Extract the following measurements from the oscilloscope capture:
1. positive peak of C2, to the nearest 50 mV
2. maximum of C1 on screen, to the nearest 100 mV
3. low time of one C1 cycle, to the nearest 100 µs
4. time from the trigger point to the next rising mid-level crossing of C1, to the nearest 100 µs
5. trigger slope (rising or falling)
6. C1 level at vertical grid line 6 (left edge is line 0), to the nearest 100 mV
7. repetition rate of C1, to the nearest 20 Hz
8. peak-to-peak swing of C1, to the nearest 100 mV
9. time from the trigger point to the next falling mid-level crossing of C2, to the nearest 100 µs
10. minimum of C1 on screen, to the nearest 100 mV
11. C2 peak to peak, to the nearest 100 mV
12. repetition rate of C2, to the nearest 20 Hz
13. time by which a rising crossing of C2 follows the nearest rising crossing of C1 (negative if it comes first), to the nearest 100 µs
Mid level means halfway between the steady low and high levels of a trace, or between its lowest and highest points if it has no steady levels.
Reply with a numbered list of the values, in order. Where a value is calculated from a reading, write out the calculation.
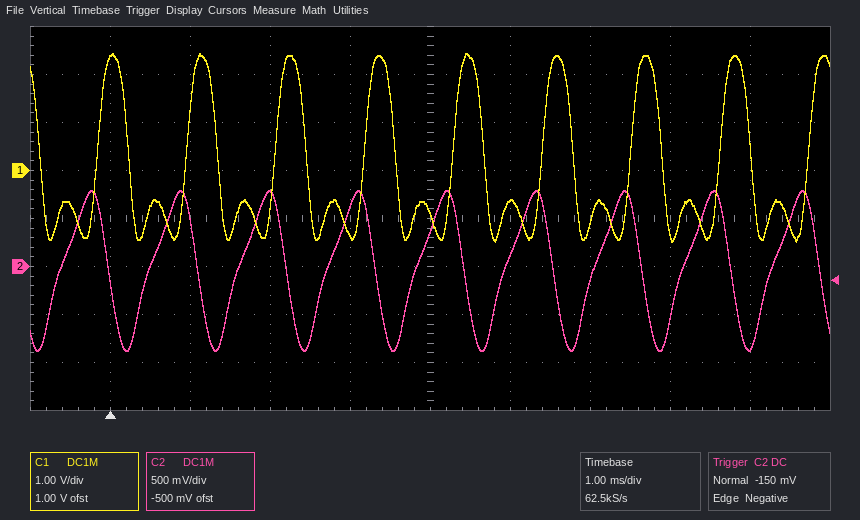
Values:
1. 800 mV
2. 2.4 V
3. 700 µs
4. 1.0 ms
5. falling
6. -700 mV
7. 900 Hz
8. 2.4 V − (-1.5 V) = 3.9 V
9. 1.1 ms
10. -1.5 V
11. 1.70 V
12. 900 Hz
13. -500 µs
